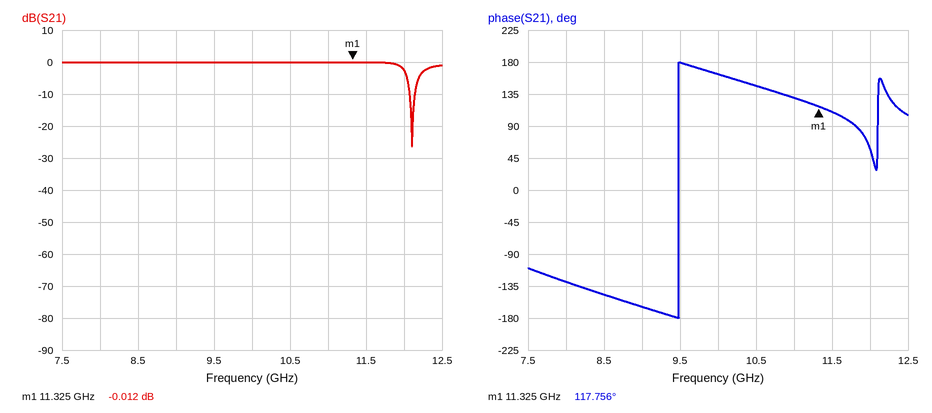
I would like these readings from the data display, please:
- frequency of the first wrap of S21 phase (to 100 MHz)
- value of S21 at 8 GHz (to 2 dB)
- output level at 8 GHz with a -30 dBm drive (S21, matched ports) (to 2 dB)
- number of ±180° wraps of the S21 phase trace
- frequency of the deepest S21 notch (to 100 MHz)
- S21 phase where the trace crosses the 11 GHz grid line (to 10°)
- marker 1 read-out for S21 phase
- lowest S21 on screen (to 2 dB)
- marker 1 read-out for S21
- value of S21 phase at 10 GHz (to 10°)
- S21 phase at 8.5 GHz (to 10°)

9.5 GHz
0 dB
-30 dBm
1
12.1 GHz
130°
117.756°
-26 dB
-0.012 dB
160°
-150°
